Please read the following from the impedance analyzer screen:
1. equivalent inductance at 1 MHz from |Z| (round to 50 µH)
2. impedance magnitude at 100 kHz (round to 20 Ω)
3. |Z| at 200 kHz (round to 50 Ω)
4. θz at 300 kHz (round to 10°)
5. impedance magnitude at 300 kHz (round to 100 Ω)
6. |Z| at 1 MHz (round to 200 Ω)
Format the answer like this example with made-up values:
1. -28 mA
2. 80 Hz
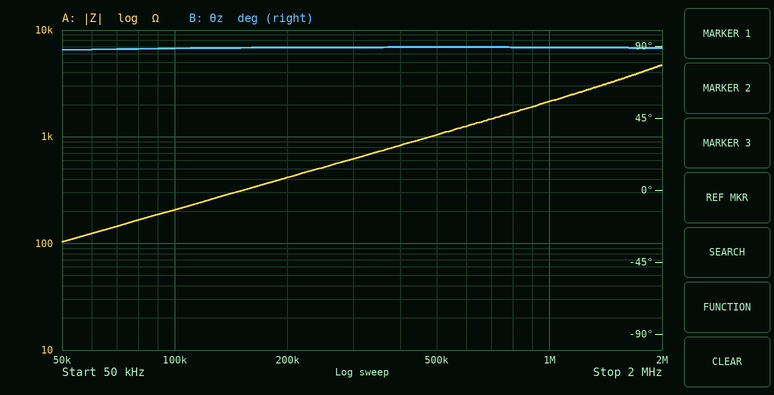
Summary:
1. 350 µH
2. 200 Ω
3. 400 Ω
4. 90°
5. 600 Ω
6. 2.2 kΩ
